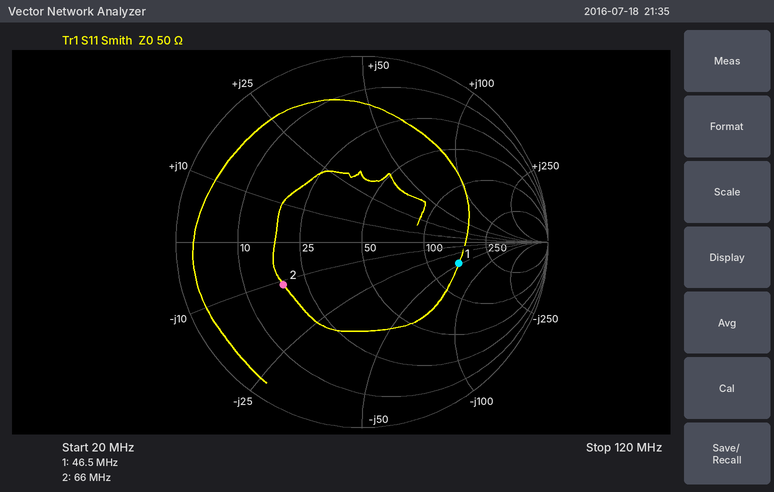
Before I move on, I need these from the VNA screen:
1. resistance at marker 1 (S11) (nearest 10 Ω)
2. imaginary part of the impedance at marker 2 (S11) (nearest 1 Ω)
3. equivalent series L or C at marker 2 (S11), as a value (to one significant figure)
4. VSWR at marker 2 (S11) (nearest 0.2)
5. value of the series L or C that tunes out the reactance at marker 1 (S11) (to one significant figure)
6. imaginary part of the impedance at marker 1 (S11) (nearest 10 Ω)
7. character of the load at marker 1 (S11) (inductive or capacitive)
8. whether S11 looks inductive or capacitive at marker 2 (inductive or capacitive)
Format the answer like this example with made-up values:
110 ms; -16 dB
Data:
150 Ω; -11 Ω; 200 pF; 2.8; 200 nH; -50 Ω; capacitive; capacitive
